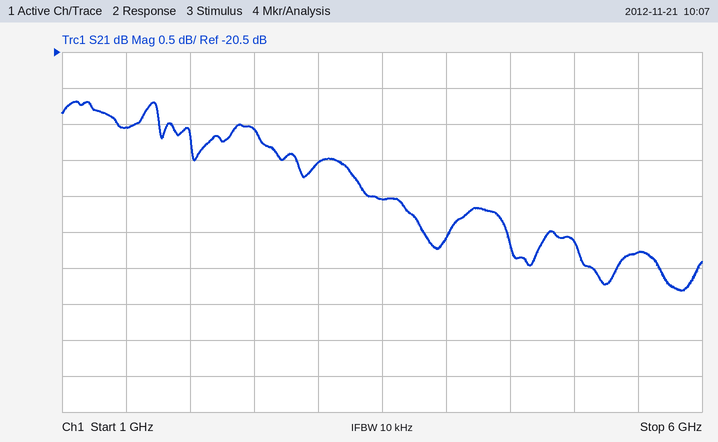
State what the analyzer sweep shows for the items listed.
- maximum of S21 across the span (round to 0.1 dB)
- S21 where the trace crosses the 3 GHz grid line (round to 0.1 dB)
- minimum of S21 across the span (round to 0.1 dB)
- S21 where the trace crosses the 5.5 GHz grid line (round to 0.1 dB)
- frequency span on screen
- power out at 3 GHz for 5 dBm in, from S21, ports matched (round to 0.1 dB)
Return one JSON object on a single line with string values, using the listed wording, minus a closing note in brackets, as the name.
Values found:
{"maximum of S21 across the span": "-21.2 dB", "S21 where the trace crosses the 3 GHz grid line": "-22.0 dB", "minimum of S21 across the span": "-23.8 dB", "S21 where the trace crosses the 5.5 GHz grid line": "-23.3 dB", "frequency span on screen": "5 GHz", "power out at 3 GHz for 5 dBm in, from S21, ports matched": "-17.0 dBm"}
